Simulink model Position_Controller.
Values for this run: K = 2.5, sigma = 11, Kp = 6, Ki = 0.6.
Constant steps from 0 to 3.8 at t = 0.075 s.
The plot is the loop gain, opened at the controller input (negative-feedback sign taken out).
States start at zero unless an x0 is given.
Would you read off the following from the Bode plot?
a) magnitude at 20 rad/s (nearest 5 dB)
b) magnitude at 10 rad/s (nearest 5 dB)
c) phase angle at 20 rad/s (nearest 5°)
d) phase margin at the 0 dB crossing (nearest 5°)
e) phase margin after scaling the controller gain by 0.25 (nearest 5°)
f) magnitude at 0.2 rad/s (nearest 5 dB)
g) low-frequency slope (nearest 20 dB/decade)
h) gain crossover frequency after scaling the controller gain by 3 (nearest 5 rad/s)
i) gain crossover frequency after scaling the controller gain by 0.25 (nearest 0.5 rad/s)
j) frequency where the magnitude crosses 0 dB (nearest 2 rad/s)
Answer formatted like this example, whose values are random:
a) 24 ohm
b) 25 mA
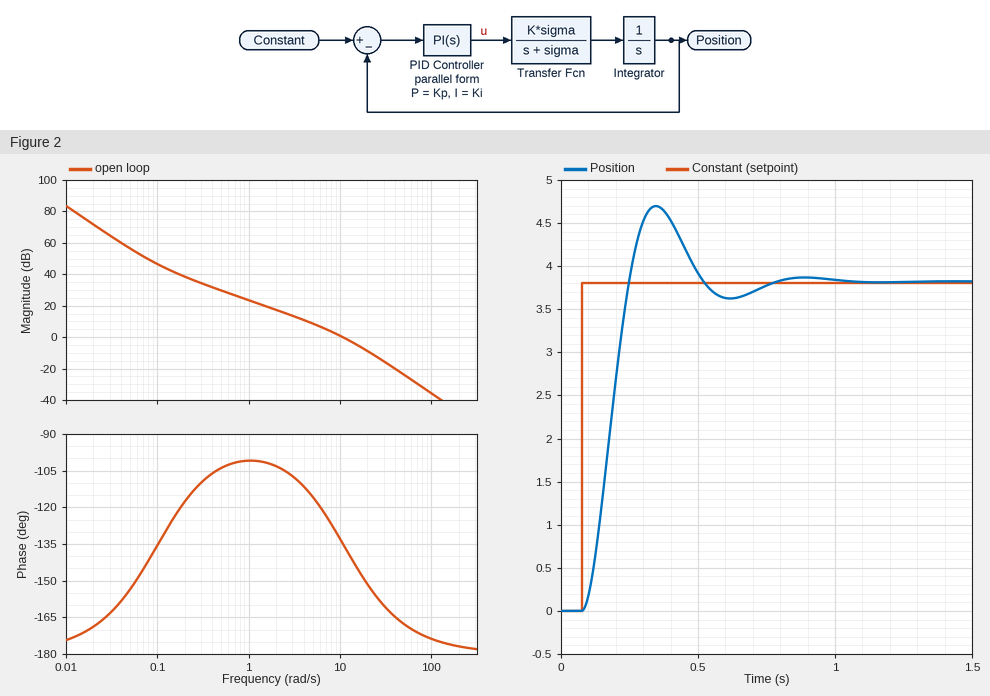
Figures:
a) -10 dB
b) 0 dB
c) -150°
d) 45°
e) 70°
f) 40 dB
g) -40 dB/decade
h) 20 rad/s
i) 3.5 rad/s
j) 10 rad/s
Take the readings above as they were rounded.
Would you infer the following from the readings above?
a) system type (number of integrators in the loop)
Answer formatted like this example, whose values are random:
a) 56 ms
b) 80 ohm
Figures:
a) 2
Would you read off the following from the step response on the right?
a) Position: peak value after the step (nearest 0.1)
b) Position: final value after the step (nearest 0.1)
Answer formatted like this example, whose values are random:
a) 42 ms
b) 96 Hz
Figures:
a) 4.7
b) 3.8
